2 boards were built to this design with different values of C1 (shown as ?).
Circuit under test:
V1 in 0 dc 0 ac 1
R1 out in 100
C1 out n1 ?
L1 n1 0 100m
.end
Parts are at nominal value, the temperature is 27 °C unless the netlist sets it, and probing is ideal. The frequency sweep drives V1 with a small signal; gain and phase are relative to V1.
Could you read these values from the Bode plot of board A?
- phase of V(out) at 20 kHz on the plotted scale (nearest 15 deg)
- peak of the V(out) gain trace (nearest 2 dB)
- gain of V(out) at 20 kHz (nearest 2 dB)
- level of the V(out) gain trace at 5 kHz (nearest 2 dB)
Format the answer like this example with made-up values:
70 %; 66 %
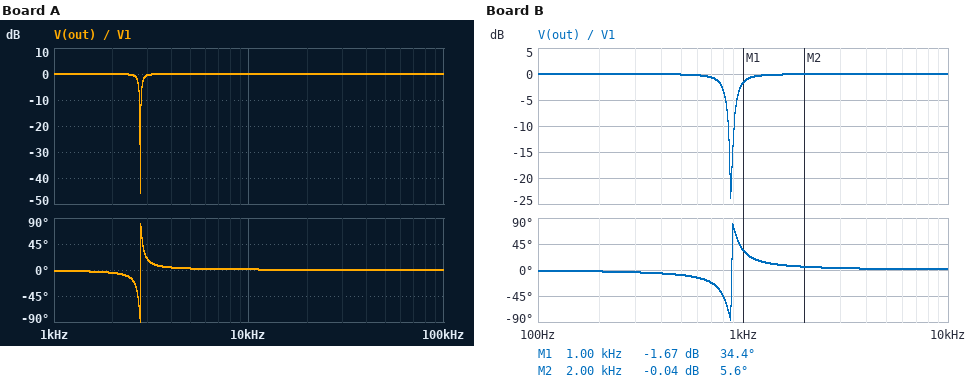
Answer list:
0 deg; 0 dB; 0 dB; 0 dB
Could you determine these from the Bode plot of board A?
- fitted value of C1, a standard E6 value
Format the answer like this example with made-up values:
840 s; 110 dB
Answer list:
33 nF
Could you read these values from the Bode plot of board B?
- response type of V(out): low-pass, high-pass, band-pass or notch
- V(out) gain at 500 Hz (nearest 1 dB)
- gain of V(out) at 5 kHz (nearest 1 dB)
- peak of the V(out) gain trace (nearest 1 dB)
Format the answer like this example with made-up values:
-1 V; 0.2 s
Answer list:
notch; 0 dB; 0 dB; 0 dB
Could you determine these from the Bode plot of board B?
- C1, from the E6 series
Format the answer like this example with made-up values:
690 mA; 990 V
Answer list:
330 nF
